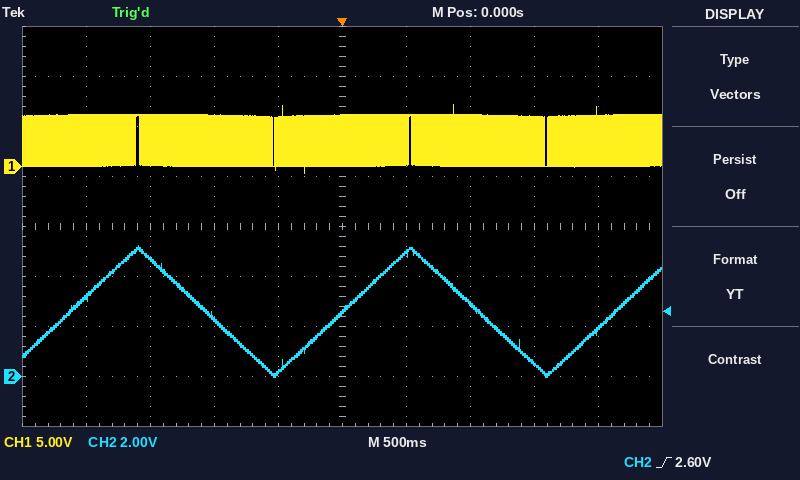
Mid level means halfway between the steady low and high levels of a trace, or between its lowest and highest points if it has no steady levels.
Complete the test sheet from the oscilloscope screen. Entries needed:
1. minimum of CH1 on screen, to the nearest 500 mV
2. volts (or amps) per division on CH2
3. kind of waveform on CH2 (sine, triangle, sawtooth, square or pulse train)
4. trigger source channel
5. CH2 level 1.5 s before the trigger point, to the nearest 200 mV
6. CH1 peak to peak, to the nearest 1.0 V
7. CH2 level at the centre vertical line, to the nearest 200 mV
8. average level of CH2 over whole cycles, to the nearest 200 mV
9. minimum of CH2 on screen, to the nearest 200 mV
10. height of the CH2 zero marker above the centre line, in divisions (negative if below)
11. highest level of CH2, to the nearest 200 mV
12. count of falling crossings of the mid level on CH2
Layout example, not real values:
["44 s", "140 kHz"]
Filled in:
["-500 mV", "2 V", "triangle", "CH2", "4.6 V", "7.0 V", "2.6 V", "2.6 V", "0.0 V", "-3.0 div", "5.2 V", "2"]
